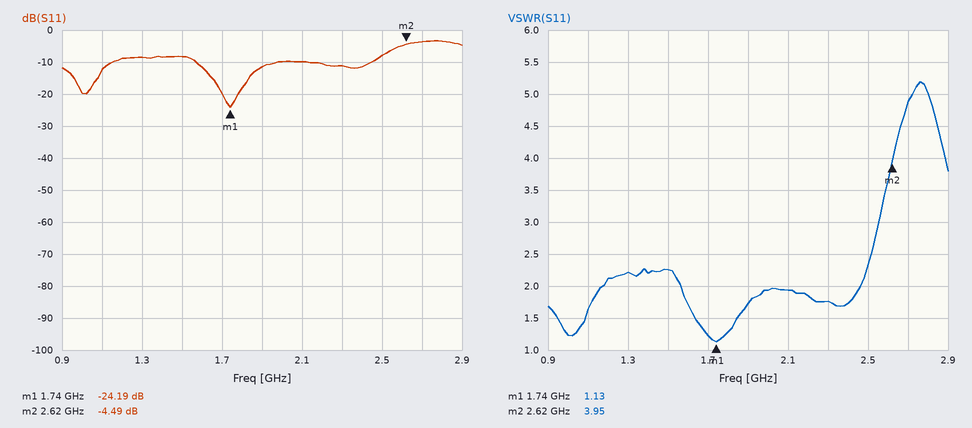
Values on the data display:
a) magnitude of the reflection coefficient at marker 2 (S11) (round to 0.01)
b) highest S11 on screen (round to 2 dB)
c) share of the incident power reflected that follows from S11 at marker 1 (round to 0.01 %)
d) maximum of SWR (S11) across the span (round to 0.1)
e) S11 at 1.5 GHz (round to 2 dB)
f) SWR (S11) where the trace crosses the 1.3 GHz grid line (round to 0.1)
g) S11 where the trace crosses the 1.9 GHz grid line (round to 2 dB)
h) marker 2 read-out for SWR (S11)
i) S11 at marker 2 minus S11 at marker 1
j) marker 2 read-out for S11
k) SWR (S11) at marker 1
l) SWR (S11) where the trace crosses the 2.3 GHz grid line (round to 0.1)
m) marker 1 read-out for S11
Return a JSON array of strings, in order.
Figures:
["0.60", "-4 dB", "0.38 %", "5.2", "-8 dB", "2.2", "-12 dB", "3.95", "19.70 dB", "-4.49 dB", "1.13", "1.8", "-24.19 dB"]
